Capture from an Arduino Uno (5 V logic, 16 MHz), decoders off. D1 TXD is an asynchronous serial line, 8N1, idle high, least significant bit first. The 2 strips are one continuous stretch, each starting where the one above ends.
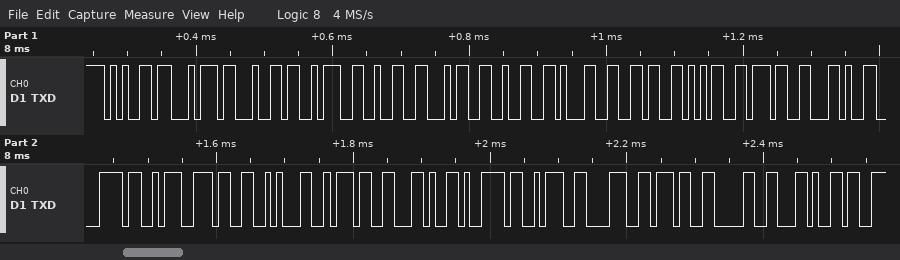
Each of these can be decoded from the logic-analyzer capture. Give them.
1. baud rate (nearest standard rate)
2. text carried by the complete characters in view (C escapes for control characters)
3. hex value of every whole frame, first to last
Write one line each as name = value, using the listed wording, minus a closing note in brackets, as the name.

baud rate = 115200 baud
text carried by the complete characters in view = "etd:2421657,x:317,y:870,"
hex value of every whole frame, first to last = 65 74 64 3A 32 34 32 31 36 35 37 2C 78 3A 33 31 37 2C 79 3A 38 37 30 2C
